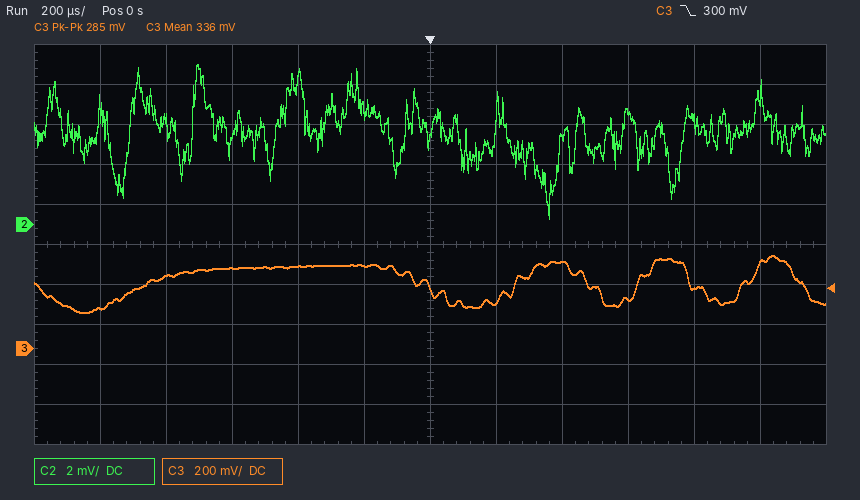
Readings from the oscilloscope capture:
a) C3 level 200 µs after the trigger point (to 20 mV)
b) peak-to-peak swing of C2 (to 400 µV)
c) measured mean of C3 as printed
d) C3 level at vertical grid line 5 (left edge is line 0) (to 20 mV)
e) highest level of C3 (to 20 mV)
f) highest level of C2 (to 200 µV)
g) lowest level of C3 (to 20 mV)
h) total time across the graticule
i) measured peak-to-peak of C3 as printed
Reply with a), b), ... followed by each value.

a) 240 mV
b) 7.6 mV
c) 336 mV
d) 420 mV
e) 460 mV
f) 8.0 mV
g) 180 mV
h) 2.4 ms
i) 285 mV
